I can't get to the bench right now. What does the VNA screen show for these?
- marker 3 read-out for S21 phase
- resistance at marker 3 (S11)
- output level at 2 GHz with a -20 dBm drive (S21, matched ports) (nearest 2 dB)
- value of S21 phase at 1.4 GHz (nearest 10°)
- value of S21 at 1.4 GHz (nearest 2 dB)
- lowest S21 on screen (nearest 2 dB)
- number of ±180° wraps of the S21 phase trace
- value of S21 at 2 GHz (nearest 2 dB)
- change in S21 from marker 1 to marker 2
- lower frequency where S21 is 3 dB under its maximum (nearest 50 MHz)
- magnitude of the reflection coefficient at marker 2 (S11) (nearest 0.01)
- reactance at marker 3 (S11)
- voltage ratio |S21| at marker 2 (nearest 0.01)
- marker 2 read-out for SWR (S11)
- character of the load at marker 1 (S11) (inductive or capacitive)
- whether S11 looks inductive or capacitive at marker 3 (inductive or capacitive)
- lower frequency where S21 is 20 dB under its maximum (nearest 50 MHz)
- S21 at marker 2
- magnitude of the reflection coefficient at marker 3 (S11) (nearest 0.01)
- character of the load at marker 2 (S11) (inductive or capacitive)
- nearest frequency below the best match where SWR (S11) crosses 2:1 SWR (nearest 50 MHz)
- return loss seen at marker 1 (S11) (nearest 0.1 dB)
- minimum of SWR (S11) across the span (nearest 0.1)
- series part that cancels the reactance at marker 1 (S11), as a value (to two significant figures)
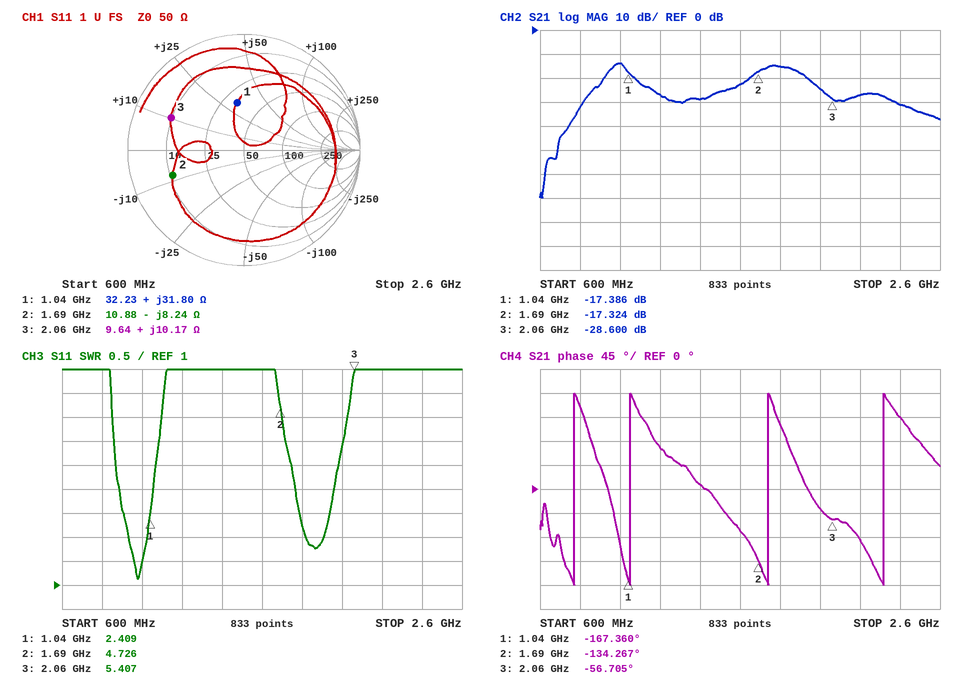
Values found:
-56.705°
9.64 Ω
-44 dBm
10°
-28 dB
-70 dB
4
-24 dB
0.062 dB
950 MHz
0.65
+10.17 Ω
0.14
4.726
inductive
inductive
800 MHz
-17.324 dB
0.69
capacitive
950 MHz
7.7 dB
1.1
4.8 pF
